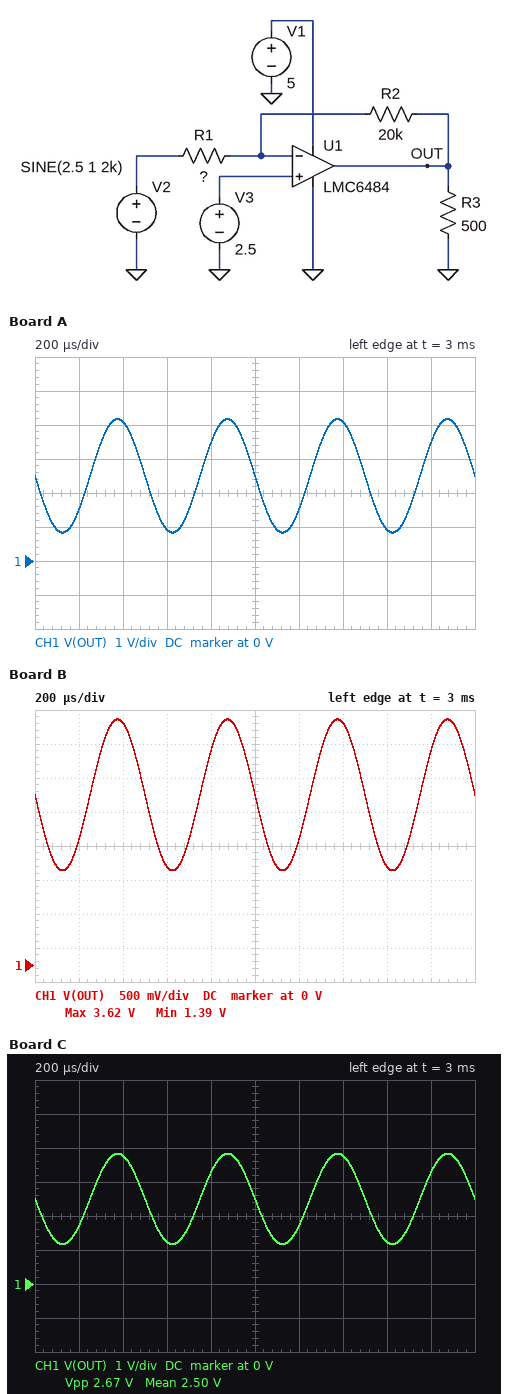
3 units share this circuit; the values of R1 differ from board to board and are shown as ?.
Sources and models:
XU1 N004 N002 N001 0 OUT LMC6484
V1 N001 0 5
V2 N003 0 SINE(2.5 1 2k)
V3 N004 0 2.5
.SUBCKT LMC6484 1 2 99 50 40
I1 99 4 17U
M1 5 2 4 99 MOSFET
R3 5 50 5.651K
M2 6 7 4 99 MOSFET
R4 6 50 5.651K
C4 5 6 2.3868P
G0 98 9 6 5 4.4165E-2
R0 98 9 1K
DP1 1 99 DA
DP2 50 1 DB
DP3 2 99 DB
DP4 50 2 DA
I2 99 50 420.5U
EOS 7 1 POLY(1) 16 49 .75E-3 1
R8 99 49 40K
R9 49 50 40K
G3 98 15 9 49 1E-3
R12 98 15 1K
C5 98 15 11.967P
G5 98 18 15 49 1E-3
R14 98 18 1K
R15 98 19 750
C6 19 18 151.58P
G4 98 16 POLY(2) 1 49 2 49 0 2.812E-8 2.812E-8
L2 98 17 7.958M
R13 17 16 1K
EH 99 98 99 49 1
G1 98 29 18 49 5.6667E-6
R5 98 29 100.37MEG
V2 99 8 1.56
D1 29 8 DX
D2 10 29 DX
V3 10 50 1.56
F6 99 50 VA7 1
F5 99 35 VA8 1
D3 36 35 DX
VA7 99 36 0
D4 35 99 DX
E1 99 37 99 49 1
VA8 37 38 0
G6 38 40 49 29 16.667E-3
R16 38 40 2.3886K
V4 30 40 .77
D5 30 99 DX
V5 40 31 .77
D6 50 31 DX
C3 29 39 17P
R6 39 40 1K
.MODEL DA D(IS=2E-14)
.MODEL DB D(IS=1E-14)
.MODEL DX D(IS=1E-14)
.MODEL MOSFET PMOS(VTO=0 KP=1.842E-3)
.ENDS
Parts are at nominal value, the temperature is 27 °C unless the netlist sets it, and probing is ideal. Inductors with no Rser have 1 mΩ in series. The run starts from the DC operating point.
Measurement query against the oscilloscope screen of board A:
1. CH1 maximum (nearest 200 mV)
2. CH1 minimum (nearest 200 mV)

4.2 V
800 mV
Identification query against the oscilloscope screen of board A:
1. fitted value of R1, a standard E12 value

12 kΩ
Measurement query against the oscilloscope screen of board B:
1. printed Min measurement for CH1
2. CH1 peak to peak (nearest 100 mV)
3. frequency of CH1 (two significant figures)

1.39 V
2.2 V
2.0 kHz
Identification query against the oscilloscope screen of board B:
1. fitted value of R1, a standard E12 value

18 kΩ
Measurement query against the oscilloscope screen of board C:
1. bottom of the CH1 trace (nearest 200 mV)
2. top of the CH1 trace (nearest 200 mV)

1.2 V
3.8 V
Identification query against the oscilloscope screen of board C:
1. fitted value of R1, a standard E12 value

15 kΩ
